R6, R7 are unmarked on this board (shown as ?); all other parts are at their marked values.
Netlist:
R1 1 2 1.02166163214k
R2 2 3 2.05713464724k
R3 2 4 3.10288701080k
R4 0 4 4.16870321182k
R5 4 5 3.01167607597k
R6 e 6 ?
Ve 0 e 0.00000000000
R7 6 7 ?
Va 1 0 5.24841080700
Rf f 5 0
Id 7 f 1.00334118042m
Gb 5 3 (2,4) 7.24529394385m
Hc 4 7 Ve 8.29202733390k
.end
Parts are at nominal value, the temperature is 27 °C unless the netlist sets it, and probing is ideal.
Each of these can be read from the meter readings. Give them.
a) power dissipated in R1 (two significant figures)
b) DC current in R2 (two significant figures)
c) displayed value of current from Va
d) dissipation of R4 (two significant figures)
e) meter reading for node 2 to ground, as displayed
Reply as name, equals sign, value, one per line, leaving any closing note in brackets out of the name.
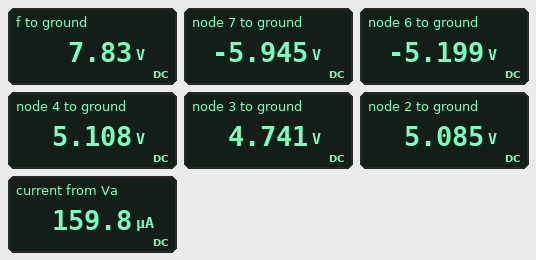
power dissipated in R1 = 26 µW
DC current in R2 = 170 µA
displayed value of current from Va = 159.8 µA
dissipation of R4 = 6.3 mW
meter reading for node 2 to ground, as displayed = 5.085 V
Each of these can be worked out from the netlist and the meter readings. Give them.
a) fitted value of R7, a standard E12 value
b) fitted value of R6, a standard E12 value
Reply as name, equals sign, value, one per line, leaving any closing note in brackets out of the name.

fitted value of R7, a standard E12 value = 560 Ω
fitted value of R6, a standard E12 value = 3.9 kΩ
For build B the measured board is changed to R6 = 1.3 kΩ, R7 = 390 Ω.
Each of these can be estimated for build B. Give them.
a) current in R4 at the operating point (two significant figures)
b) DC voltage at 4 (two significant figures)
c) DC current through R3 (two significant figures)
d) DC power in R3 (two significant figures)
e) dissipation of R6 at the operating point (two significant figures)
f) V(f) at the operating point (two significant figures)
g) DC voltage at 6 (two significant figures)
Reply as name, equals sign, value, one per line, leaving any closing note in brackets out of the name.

current in R4 at the operating point = 1.1 mA
DC voltage at 4 = 4.6 V
DC current through R3 = 33 µA
DC power in R3 = 3.4 µW
dissipation of R6 at the operating point = 640 µW
V(f) at the operating point = 9.0 V
DC voltage at 6 = -910 mV
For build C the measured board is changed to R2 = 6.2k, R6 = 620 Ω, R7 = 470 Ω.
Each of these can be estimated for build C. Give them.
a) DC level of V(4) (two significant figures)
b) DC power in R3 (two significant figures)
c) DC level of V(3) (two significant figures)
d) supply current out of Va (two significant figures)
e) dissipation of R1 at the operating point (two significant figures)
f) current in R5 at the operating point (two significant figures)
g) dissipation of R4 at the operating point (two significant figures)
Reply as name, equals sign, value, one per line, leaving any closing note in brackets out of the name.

DC level of V(4) = 4.6 V
DC power in R3 = 4.0 µW
DC level of V(3) = -550 mV
supply current out of Va = 770 µA
dissipation of R1 at the operating point = 610 µW
current in R5 at the operating point = 1.5 mA
dissipation of R4 at the operating point = 5.0 mW
